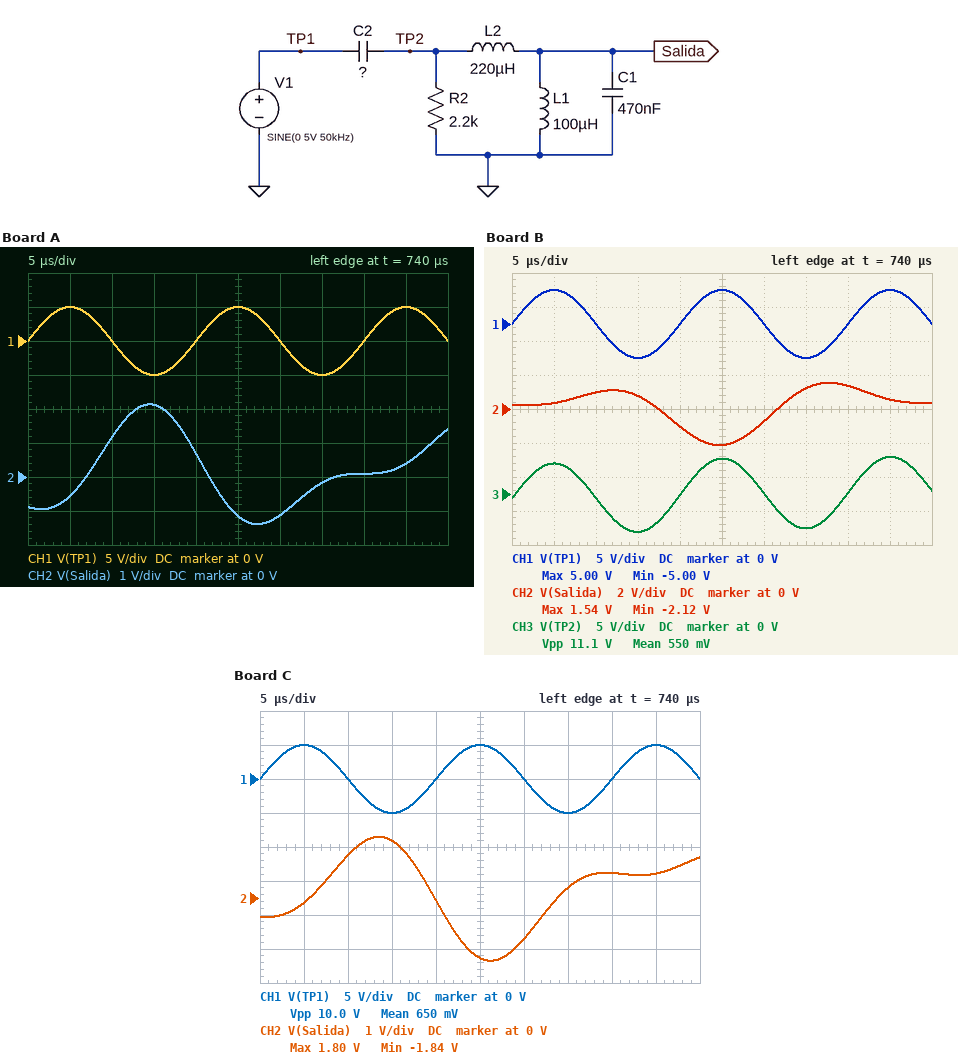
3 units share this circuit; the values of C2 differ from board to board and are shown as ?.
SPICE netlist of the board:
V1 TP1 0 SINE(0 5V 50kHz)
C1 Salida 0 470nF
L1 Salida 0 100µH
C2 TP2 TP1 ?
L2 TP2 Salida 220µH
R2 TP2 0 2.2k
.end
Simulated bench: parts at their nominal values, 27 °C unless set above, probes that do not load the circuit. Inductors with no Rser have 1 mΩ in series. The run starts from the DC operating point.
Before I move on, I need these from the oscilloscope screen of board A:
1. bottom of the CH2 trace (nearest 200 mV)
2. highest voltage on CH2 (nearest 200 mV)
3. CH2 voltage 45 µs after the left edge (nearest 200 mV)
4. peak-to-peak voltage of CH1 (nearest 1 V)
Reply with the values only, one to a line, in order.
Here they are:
-1.4 V
2.2 V
400 mV
10 V
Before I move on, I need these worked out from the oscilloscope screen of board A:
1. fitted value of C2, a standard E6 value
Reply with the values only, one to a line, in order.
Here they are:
3.3 µF
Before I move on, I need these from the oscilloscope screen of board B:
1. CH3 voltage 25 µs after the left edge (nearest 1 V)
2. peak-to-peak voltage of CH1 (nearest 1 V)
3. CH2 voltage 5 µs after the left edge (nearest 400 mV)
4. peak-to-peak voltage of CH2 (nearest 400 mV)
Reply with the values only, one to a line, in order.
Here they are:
5 V
10 V
400 mV
3.6 V
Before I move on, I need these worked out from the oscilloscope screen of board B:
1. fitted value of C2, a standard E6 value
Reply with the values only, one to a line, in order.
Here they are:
1.5 µF
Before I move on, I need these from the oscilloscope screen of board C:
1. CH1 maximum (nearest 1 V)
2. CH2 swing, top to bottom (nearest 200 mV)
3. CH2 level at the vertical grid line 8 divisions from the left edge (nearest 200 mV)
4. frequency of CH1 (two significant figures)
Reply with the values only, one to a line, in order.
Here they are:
5 V
3.6 V
800 mV
50 kHz
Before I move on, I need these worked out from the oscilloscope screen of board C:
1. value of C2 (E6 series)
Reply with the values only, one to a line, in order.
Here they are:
2.2 µF
